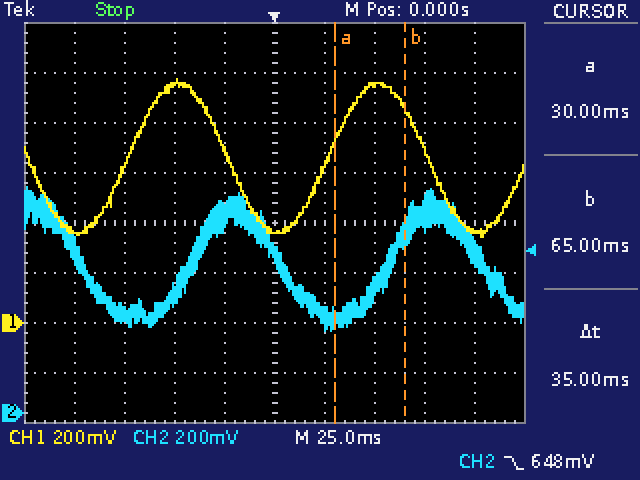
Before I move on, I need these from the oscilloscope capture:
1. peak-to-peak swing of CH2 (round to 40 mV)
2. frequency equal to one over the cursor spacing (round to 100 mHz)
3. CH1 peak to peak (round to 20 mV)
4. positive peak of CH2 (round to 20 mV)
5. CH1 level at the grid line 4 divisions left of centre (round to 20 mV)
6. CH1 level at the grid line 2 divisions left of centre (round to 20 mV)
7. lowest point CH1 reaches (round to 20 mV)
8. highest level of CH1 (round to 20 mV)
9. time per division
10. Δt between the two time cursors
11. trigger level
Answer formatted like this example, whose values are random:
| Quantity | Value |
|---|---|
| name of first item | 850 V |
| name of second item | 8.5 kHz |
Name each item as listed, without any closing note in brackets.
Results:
| Quantity | Value |
|---|---|
| peak-to-peak swing of CH2 | 560 mV |
| frequency equal to one over the cursor spacing | 28.6 Hz |
| CH1 peak to peak | 640 mV |
| positive peak of CH2 | 900 mV |
| CH1 level at the grid line 4 divisions left of centre | 360 mV |
| CH1 level at the grid line 2 divisions left of centre | 960 mV |
| lowest point CH1 reaches | 340 mV |
| highest level of CH1 | 980 mV |
| time per division | 25 ms |
| Δt between the two time cursors | 35 ms |
| trigger level | 648 mV |
